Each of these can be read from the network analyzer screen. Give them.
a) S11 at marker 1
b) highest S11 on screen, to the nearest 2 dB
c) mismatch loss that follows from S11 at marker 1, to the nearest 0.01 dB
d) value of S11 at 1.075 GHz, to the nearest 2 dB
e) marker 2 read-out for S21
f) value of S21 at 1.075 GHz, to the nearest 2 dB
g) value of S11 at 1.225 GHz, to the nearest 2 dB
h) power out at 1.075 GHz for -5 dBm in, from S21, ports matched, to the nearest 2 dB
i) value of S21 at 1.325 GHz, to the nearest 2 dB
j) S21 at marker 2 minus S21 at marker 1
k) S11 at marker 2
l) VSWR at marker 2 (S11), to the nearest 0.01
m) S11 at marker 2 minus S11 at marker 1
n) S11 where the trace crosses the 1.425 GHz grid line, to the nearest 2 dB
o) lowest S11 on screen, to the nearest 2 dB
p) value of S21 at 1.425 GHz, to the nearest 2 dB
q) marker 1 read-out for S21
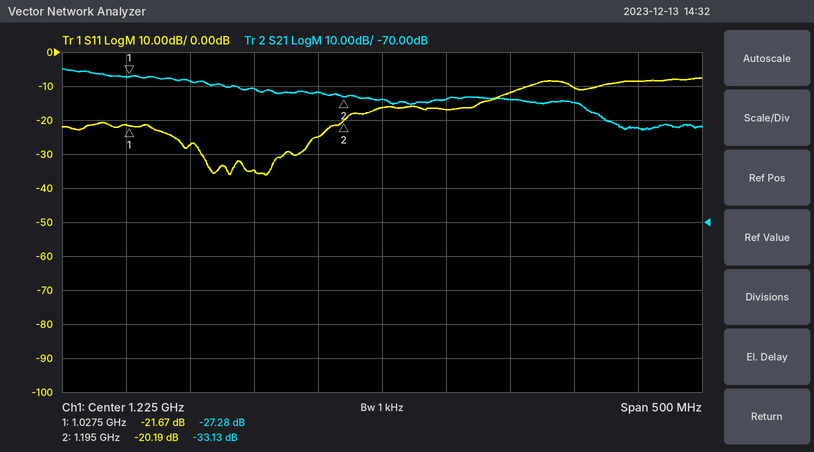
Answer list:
-21.67 dB
-8 dB
0.03 dB
-28 dB
-33.13 dB
-28 dB
-16 dB
-34 dBm
-34 dB
-5.85 dB
-20.19 dB
1.22
1.48 dB
-8 dB
-36 dB
-42 dB
-27.28 dB
